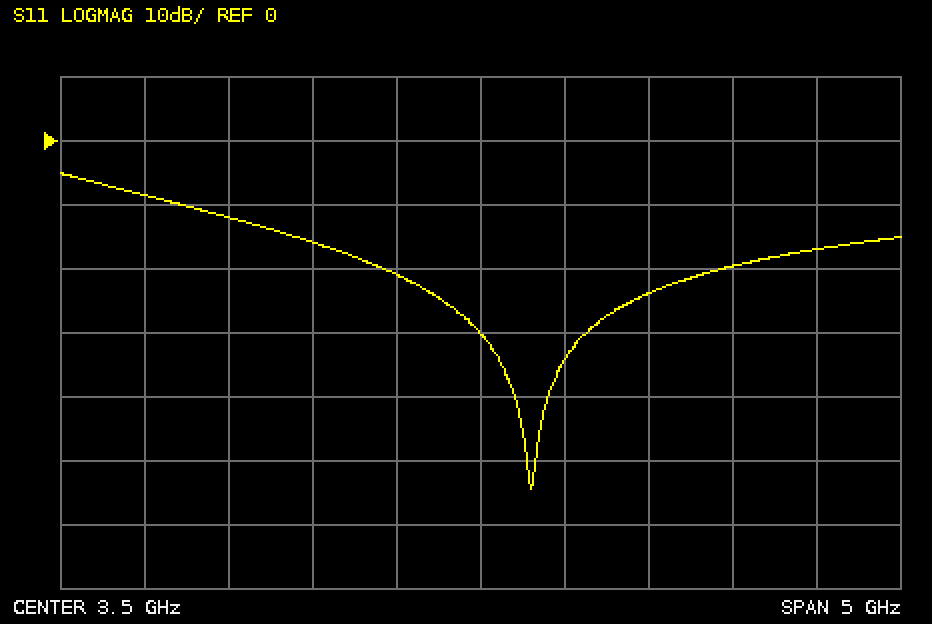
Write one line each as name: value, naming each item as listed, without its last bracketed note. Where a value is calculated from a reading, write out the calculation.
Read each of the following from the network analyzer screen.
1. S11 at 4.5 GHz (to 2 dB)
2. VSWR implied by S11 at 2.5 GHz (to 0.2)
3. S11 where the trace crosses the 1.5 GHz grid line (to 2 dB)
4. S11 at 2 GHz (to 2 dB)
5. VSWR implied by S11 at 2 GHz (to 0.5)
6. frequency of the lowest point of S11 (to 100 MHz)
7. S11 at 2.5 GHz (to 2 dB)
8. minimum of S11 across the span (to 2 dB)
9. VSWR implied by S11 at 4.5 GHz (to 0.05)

S11 at 4.5 GHz: -24 dB
VSWR implied by S11 at 2.5 GHz: |Γ| = 10^(-16/20) = 0.1585; VSWR = (1 + 0.1585)/(1 − 0.1585) ≈ 1.4
S11 where the trace crosses the 1.5 GHz grid line: -8 dB
S11 at 2 GHz: -12 dB
VSWR implied by S11 at 2 GHz: |Γ| = 10^(-12/20) = 0.2512; VSWR = (1 + 0.2512)/(1 − 0.2512) ≈ 1.67, so 1.5 to the nearest 0.5
frequency of the lowest point of S11: 3.8 GHz
S11 at 2.5 GHz: -16 dB
minimum of S11 across the span: -54 dB
VSWR implied by S11 at 4.5 GHz: |Γ| = 10^(-24/20) = 0.0631; VSWR = (1 + 0.0631)/(1 − 0.0631) ≈ 1.13, so 1.15 to the nearest 0.05
